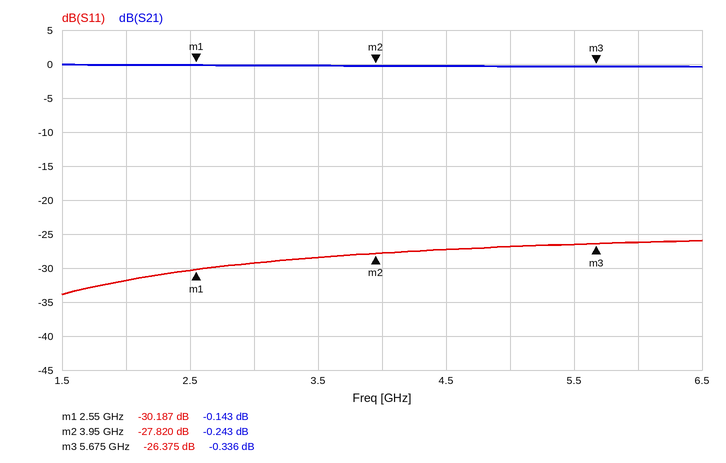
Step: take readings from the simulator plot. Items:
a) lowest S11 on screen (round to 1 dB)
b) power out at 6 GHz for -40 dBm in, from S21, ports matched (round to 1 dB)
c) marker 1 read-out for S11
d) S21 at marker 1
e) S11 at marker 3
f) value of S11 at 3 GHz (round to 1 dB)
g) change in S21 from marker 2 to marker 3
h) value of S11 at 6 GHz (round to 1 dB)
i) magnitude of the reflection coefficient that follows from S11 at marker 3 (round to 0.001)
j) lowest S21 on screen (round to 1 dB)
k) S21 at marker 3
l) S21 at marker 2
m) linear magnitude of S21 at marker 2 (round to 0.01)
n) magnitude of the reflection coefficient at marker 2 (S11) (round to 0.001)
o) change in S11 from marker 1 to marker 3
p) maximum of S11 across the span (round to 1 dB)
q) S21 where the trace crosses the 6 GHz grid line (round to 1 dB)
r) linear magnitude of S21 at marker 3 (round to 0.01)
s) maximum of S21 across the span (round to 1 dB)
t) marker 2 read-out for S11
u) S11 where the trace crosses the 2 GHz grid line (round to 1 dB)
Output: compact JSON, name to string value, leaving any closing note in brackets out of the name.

{"lowest S11 on screen": "-34 dB", "power out at 6 GHz for -40 dBm in, from S21, ports matched": "-40 dBm", "marker 1 read-out for S11": "-30.187 dB", "S21 at marker 1": "-0.143 dB", "S11 at marker 3": "-26.375 dB", "value of S11 at 3 GHz": "-29 dB", "change in S21 from marker 2 to marker 3": "-0.093 dB", "value of S11 at 6 GHz": "-26 dB", "magnitude of the reflection coefficient that follows from S11 at marker 3": "0.048", "lowest S21 on screen": "0 dB", "S21 at marker 3": "-0.336 dB", "S21 at marker 2": "-0.243 dB", "linear magnitude of S21 at marker 2": "0.97", "magnitude of the reflection coefficient at marker 2 (S11)": "0.041", "change in S11 from marker 1 to marker 3": "3.812 dB", "maximum of S11 across the span": "-26 dB", "S21 where the trace crosses the 6 GHz grid line": "0 dB", "linear magnitude of S21 at marker 3": "0.96", "maximum of S21 across the span": "0 dB", "marker 2 read-out for S11": "-27.820 dB", "S11 where the trace crosses the 2 GHz grid line": "-32 dB"}
